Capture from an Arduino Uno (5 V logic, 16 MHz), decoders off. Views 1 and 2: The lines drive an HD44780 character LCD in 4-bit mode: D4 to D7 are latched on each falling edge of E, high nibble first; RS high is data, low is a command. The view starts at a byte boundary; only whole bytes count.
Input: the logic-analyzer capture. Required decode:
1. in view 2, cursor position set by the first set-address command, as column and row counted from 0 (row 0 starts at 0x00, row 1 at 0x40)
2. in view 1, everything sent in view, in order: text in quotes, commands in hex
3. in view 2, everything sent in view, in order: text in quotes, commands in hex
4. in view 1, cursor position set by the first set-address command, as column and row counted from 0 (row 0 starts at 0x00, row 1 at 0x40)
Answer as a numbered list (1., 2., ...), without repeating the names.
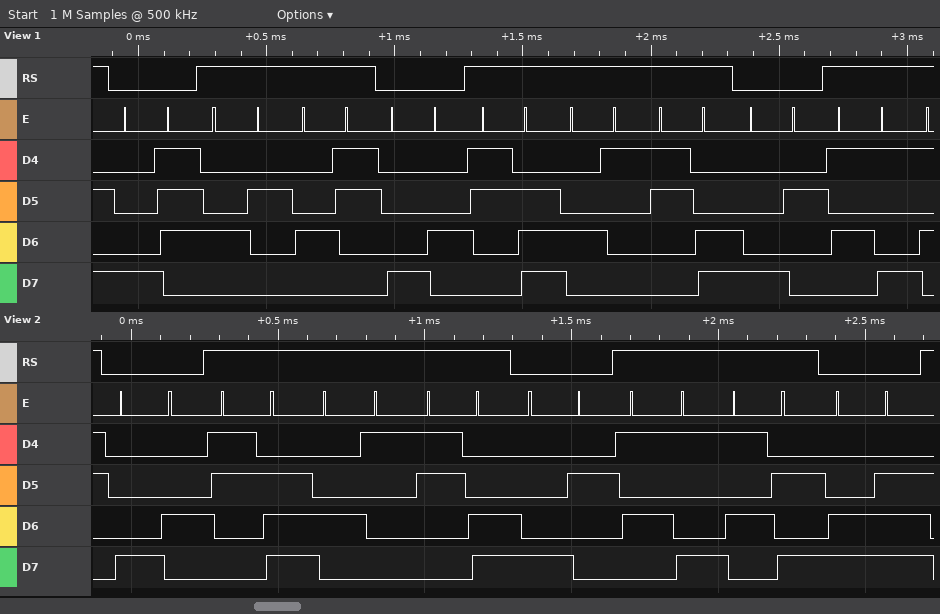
1. column 4, row 0
2. 0x87 "BC" 0x84 ">A<" 0x82 "Y"
3. 0x84 ">A<" 0x82 "YZ" 0xCE
4. column 7, row 0
